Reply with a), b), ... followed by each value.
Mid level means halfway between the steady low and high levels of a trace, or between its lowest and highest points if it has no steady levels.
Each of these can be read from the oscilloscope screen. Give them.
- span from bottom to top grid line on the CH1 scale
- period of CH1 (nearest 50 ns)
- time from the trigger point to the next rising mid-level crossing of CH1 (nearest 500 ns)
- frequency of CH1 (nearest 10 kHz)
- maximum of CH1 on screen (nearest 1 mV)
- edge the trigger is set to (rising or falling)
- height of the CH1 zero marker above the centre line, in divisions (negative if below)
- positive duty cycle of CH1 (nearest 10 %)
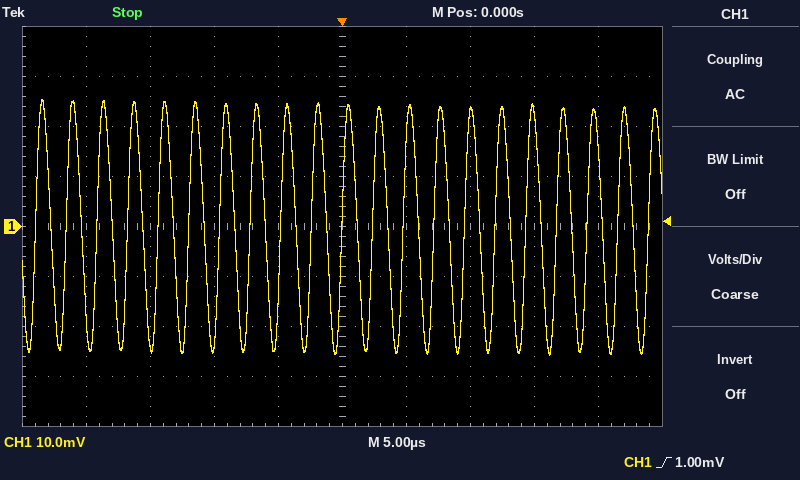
a) 80 mV
b) 2.40 µs
c) 2.5 µs
d) 420 kHz
e) 25 mV
f) rising
g) 0.0 div
h) 50 %
